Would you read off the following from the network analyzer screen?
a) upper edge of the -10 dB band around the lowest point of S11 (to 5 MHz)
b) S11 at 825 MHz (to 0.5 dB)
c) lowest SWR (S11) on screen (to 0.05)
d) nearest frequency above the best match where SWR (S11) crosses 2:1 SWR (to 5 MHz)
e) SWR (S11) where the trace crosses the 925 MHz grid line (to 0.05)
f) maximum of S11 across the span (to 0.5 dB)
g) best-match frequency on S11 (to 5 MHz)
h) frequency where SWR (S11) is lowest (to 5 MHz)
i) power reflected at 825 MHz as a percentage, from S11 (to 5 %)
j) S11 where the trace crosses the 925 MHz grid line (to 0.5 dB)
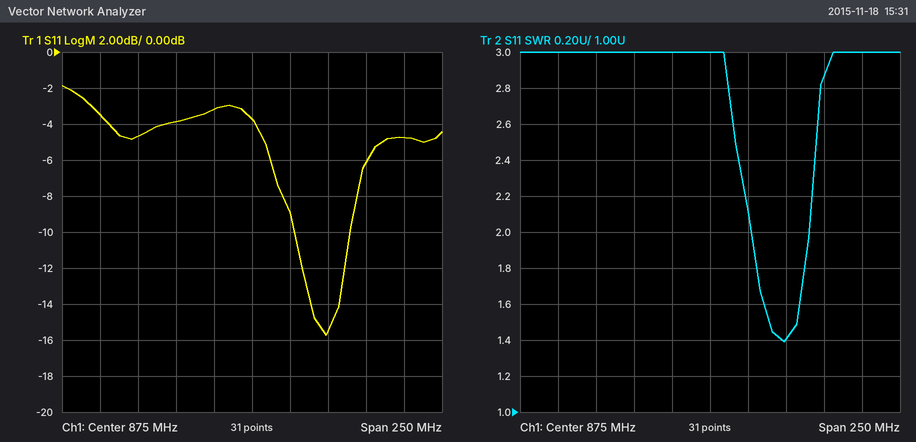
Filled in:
940 MHz
-4.0 dB
1.40
940 MHz
1.40
-2.0 dB
925 MHz
925 MHz
40 %
-15.5 dB
